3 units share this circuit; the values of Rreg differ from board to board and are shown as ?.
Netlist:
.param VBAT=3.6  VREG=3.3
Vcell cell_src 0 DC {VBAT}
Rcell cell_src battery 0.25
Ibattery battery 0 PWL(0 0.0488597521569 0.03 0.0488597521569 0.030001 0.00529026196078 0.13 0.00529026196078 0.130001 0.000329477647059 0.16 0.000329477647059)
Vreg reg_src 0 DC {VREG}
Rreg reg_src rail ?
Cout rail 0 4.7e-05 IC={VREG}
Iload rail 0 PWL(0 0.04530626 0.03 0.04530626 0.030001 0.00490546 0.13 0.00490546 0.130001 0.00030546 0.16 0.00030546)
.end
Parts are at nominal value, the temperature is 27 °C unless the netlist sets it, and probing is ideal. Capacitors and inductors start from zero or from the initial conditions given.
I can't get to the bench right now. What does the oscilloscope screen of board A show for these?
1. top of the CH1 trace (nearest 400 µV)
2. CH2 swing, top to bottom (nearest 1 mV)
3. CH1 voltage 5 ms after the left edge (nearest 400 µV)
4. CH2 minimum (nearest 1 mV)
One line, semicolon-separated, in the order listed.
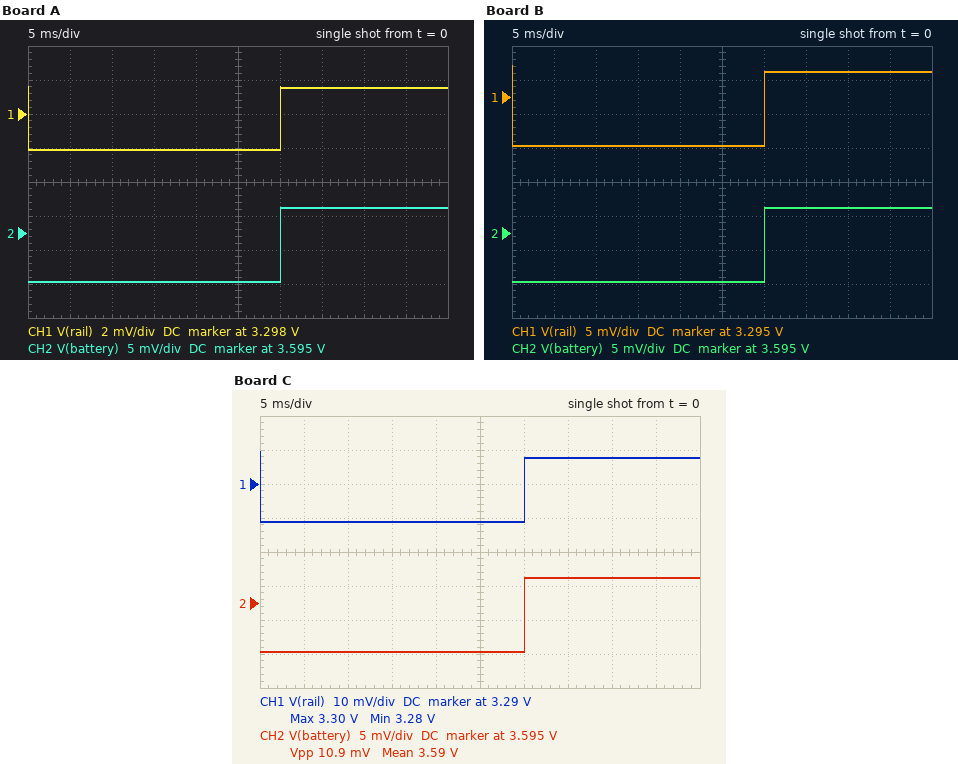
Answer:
3.2996 V; 11 mV; 3.2960 V; 3.588 V
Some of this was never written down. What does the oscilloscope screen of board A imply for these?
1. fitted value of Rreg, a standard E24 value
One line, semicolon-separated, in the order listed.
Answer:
0.091 Ω
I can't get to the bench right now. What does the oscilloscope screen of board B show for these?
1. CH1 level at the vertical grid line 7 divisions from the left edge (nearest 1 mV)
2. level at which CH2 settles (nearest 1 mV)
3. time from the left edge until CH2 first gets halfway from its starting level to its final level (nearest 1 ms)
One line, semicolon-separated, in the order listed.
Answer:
3.299 V; 3.599 V; 30 ms
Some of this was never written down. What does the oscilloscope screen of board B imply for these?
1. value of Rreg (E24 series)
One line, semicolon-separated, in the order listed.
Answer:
0.27 Ω
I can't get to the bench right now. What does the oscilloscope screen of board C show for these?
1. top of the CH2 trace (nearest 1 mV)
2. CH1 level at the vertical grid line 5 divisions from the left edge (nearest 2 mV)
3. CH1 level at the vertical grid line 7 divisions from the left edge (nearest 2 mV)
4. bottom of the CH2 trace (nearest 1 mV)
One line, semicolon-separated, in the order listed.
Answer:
3.599 V; 3.278 V; 3.298 V; 3.588 V
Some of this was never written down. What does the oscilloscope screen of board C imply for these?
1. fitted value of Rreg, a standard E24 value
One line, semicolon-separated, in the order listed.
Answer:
0.47 Ω
